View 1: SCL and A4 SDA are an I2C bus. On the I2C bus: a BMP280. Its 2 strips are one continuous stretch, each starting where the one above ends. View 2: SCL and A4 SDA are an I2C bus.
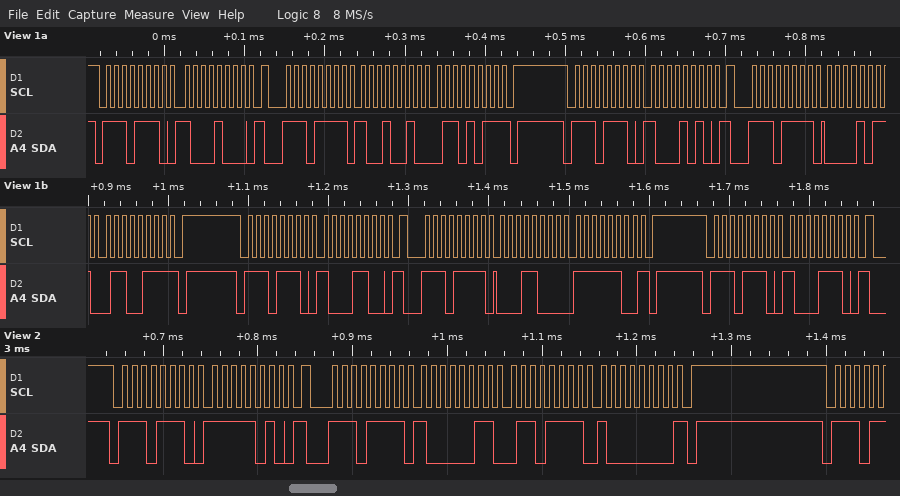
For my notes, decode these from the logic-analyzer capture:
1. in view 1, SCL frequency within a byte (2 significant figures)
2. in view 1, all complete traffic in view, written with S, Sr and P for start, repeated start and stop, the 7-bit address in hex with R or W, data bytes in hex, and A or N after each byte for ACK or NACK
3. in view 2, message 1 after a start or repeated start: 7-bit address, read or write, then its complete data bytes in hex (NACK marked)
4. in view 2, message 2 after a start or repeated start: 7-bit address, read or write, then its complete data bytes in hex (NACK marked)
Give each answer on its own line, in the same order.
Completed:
100 kHz
S 77W A 88 A Sr 77R A 92 A 6B N P S 77W A 8A A Sr 77R A 0B A 67 N P S 77W A 8C A Sr 77R A 18 A FC N P S 77W A 8E A
0x77 write: FA
0x77 read: 83 6F 80 NACK
